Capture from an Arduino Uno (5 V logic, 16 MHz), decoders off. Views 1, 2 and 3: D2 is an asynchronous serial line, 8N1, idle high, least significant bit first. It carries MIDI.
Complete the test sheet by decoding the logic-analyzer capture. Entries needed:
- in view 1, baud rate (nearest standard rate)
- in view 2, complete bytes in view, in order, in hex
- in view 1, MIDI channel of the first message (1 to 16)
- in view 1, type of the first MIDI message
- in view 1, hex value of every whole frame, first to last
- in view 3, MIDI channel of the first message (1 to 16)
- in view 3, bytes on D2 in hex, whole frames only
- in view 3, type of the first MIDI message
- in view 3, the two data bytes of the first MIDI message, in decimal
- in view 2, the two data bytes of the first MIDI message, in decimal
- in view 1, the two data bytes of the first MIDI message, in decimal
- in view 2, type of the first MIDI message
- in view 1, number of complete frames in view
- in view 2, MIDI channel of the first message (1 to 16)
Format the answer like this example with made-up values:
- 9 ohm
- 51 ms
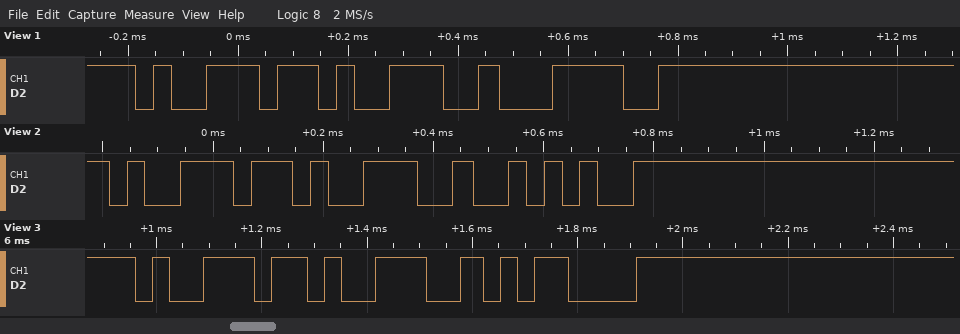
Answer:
- 31250 baud
- 0xB9 0x39 0x2A
- 10
- Control Change
- B9 39 3C
- 10
- B9 39 0D
- Control Change
- 57, 13
- 57, 42
- 57, 60
- Control Change
- 3
- 10
